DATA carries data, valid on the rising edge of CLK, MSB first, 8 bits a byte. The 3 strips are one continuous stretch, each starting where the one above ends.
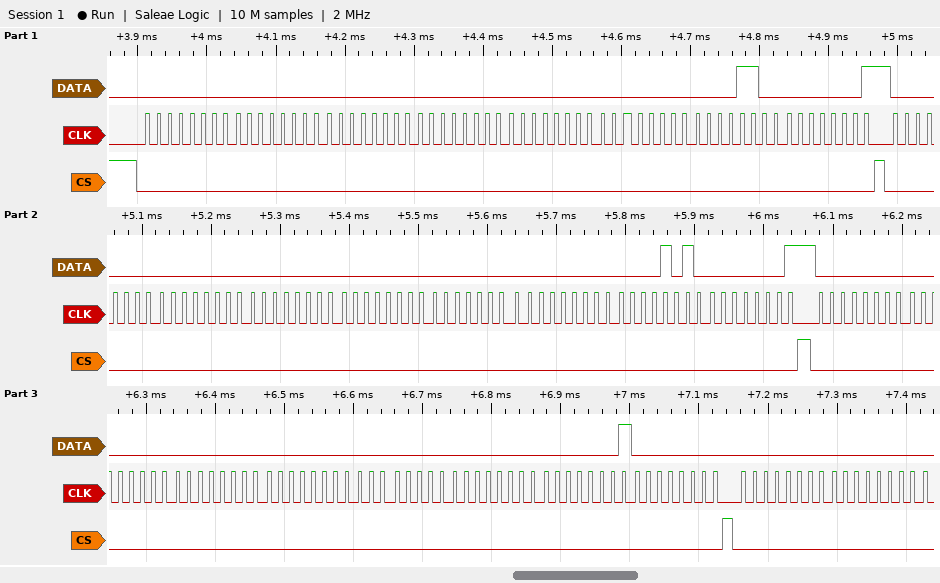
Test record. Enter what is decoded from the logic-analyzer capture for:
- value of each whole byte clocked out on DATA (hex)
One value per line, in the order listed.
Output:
0x00 0x00 0x00 0x00 0x00 0x00 0x0C 0x01 0x00 0x00 0x00 0x00 0x00 0x00 0x0A 0x01 0x00 0x00 0x00 0x00 0x00 0x00 0x01 0x00 0x00 0x00
